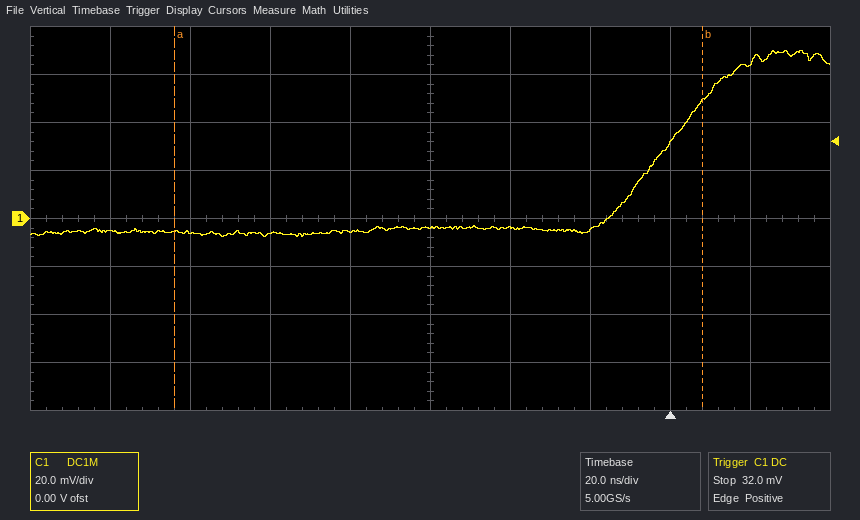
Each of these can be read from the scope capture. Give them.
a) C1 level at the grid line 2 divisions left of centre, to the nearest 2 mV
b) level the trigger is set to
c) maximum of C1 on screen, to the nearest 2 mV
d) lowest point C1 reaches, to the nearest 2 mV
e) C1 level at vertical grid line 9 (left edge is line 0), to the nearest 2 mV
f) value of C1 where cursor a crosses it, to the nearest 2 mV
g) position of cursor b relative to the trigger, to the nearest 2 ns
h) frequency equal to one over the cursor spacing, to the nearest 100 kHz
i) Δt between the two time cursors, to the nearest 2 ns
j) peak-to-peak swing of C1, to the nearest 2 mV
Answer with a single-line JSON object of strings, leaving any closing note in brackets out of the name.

{"C1 level at the grid line 2 divisions left of centre, to the nearest 2 mV": "-6 mV", "level the trigger is set to": "32.0 mV", "maximum of C1 on screen, to the nearest 2 mV": "70 mV", "lowest point C1 reaches, to the nearest 2 mV": "-8 mV", "C1 level at vertical grid line 9 (left edge is line 0), to the nearest 2 mV": "66 mV", "value of C1 where cursor a crosses it, to the nearest 2 mV": "-6 mV", "position of cursor b relative to the trigger, to the nearest 2 ns": "+8 ns", "frequency equal to one over the cursor spacing, to the nearest 100 kHz": "7.6 MHz", "Δt between the two time cursors, to the nearest 2 ns": "132 ns", "peak-to-peak swing of C1, to the nearest 2 mV": "78 mV"}
